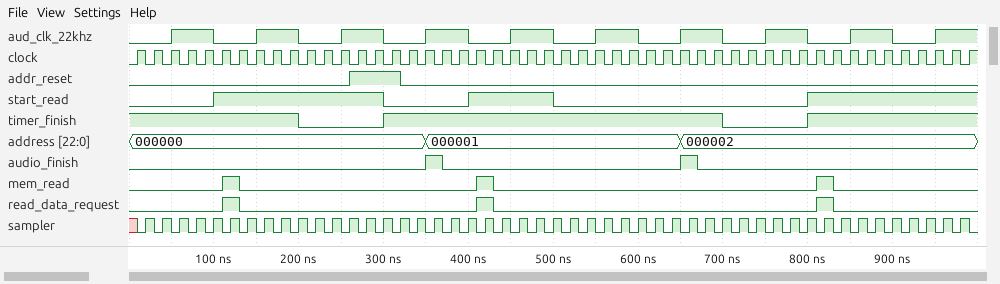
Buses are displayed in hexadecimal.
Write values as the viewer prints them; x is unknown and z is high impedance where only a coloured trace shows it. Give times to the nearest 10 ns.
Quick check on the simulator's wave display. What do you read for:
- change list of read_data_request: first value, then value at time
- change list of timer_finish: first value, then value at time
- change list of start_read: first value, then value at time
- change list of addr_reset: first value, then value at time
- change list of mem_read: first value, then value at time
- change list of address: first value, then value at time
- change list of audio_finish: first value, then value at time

0, 1 at 110 ns, 0 at 130 ns, 1 at 410 ns, 0 at 430 ns, 1 at 810 ns, 0 at 830 ns
1, 0 at 200 ns, 1 at 300 ns, 0 at 700 ns, 1 at 800 ns
0, 1 at 100 ns, 0 at 300 ns, 1 at 400 ns, 0 at 500 ns, 1 at 800 ns
0, 1 at 260 ns, 0 at 320 ns
0, 1 at 110 ns, 0 at 130 ns, 1 at 410 ns, 0 at 430 ns, 1 at 810 ns, 0 at 830 ns
000000, 000001 at 350 ns, 000002 at 650 ns
0, 1 at 350 ns, 0 at 370 ns, 1 at 650 ns, 0 at 670 ns
